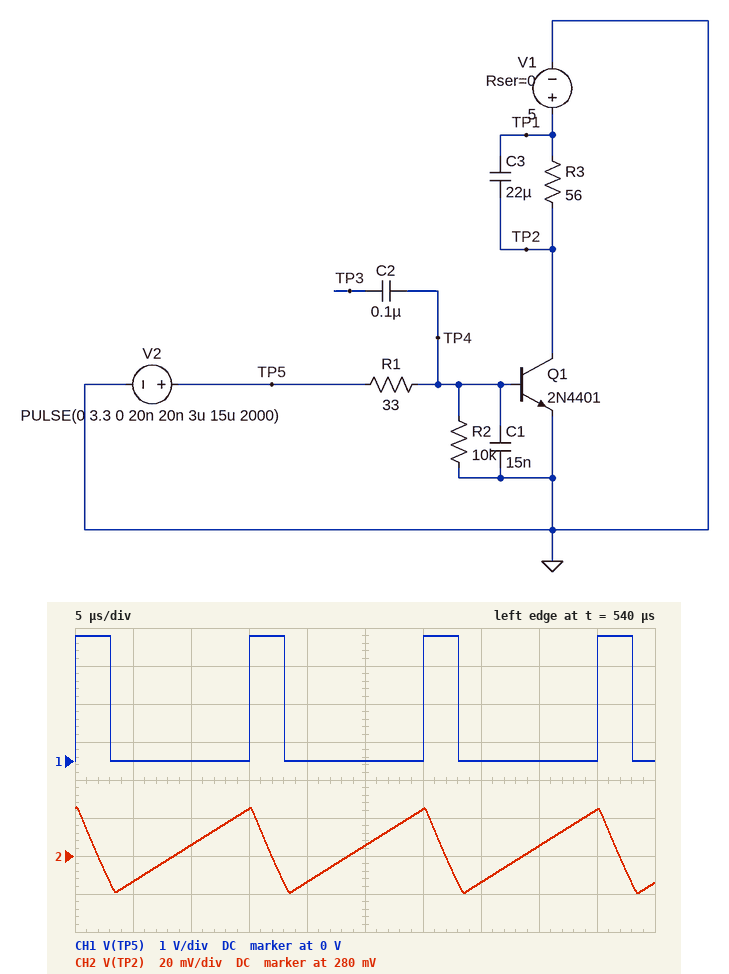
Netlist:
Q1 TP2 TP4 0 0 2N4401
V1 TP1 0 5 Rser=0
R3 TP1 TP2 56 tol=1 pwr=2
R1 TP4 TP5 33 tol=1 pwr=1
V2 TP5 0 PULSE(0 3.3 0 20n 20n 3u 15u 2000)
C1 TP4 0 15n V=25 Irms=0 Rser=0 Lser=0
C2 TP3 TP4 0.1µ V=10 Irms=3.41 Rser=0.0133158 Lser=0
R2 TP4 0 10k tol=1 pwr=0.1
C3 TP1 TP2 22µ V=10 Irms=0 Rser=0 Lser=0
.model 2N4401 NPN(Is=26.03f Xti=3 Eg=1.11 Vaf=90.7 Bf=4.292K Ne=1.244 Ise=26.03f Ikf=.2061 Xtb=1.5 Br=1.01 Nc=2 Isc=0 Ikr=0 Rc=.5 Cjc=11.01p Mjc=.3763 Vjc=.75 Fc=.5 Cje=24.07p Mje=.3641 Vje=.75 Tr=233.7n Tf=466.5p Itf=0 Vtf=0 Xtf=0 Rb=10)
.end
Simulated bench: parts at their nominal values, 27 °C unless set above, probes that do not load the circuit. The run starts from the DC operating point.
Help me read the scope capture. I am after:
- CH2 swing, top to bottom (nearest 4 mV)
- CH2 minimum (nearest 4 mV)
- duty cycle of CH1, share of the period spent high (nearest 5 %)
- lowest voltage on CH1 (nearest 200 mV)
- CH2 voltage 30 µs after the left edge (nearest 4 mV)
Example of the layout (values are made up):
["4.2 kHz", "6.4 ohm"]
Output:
["44 mV", "260 mV", "20 %", "0 V", "304 mV"]
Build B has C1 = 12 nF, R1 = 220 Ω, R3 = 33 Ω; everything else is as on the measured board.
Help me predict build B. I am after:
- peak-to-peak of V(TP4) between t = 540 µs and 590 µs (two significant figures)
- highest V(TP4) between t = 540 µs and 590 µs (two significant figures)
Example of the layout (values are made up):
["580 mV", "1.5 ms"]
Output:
["950 mV", "960 mV"]
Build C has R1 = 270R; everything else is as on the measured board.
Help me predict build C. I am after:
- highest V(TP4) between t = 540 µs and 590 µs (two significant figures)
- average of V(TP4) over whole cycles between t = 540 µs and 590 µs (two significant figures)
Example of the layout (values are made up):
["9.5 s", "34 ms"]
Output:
["940 mV", "370 mV"]
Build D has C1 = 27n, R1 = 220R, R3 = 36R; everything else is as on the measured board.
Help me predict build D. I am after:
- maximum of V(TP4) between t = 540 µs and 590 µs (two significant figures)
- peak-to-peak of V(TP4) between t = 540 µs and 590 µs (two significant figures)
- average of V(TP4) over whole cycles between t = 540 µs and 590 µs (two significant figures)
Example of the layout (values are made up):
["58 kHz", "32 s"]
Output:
["960 mV", "850 mV", "440 mV"]
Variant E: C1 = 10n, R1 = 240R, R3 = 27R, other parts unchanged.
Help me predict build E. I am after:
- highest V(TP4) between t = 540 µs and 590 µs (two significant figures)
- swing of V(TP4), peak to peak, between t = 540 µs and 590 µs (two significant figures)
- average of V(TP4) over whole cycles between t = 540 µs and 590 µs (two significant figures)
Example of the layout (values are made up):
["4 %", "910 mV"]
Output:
["950 mV", "940 mV", "300 mV"]
